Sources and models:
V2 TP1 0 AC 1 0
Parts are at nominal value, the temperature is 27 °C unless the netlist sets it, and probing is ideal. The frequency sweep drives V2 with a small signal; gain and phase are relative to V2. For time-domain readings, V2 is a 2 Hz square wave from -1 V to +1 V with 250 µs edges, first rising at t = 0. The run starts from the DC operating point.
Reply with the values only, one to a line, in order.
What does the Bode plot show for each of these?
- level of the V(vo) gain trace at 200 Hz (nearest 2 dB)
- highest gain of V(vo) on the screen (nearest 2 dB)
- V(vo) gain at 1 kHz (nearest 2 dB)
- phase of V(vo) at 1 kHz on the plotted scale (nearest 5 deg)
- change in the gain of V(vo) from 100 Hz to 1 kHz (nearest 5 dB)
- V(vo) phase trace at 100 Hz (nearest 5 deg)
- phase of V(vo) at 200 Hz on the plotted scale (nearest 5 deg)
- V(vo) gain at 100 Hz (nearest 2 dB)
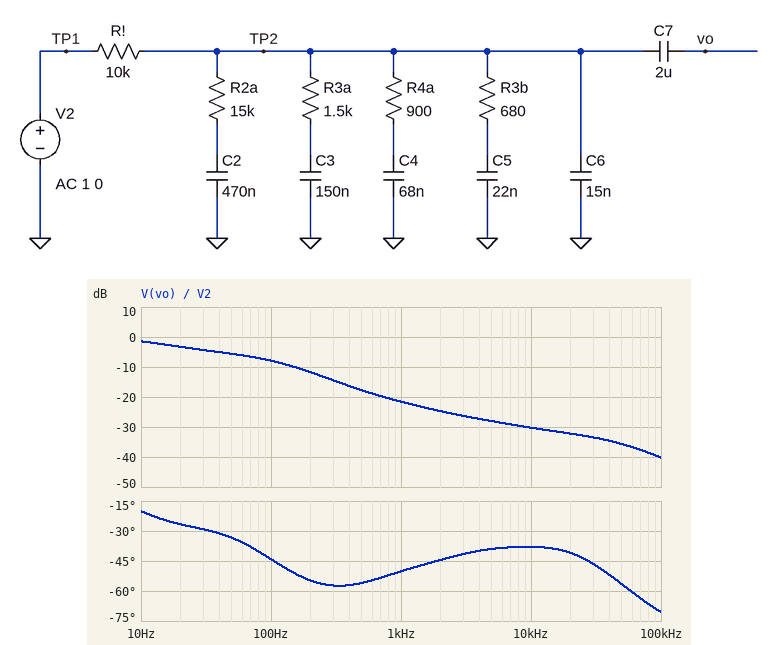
-12 dB
-2 dB
-22 dB
-50 deg
-15 dB
-45 deg
-55 deg
-8 dB
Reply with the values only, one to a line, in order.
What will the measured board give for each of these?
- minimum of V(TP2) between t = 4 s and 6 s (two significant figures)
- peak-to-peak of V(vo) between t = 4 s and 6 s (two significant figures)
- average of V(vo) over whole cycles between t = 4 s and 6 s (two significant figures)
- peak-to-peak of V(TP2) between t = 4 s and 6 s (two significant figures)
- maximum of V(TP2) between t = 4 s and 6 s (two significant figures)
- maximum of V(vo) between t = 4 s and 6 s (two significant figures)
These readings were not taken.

-1.0 V
2.0 V
1.0 V
2.0 V
1.0 V
2.0 V
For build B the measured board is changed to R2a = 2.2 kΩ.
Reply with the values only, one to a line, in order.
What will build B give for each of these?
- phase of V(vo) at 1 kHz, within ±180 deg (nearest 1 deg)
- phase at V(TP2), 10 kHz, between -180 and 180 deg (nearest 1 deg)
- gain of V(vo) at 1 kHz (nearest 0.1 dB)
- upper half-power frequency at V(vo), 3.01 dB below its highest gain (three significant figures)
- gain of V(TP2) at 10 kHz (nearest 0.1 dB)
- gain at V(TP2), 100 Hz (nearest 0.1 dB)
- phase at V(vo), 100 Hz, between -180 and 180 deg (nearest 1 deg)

-41 deg
-34 deg
-23.6 dB
20.2 Hz
-31.0 dB
-12.9 dB
-56 deg
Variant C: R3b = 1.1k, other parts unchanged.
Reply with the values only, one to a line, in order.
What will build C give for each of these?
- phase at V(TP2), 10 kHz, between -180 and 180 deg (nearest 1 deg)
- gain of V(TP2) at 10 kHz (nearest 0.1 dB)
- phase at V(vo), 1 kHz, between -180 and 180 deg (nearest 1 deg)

-34 deg
-29.6 dB
-50 deg
